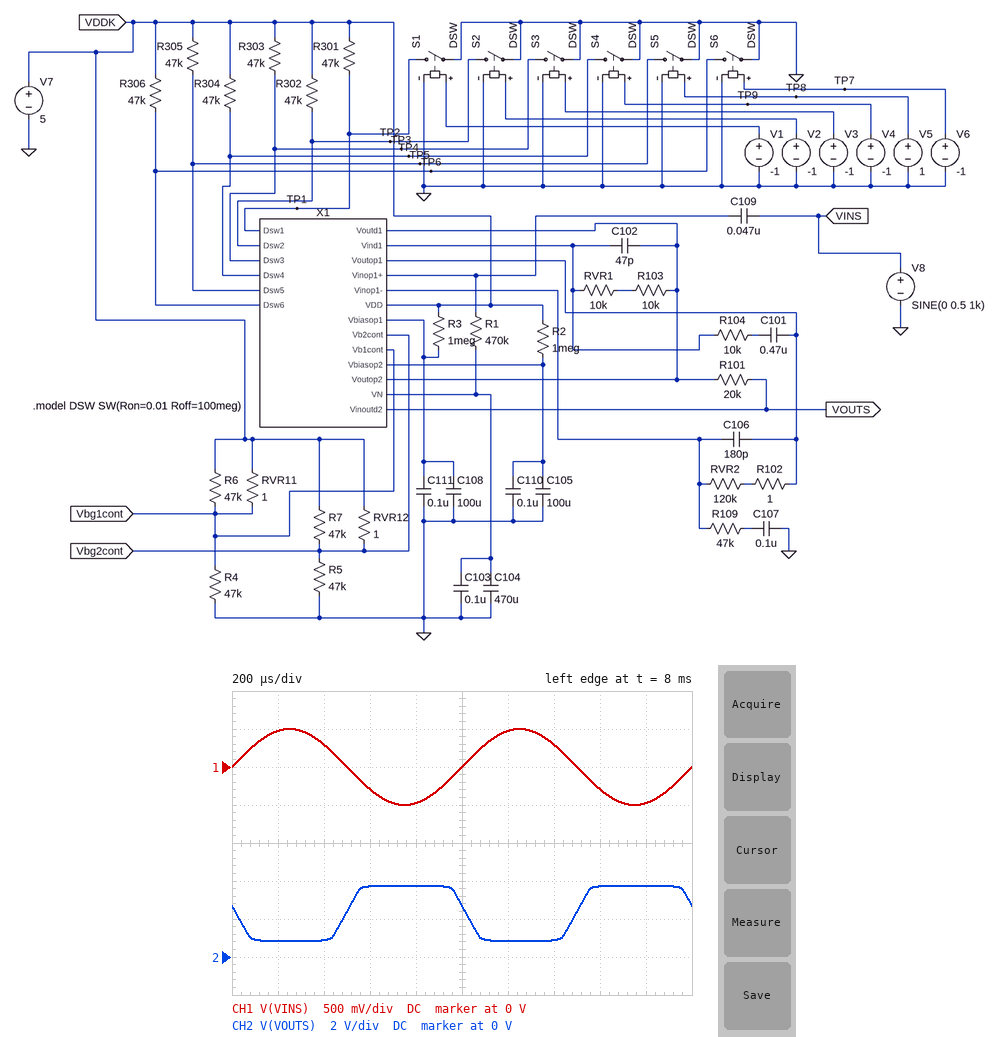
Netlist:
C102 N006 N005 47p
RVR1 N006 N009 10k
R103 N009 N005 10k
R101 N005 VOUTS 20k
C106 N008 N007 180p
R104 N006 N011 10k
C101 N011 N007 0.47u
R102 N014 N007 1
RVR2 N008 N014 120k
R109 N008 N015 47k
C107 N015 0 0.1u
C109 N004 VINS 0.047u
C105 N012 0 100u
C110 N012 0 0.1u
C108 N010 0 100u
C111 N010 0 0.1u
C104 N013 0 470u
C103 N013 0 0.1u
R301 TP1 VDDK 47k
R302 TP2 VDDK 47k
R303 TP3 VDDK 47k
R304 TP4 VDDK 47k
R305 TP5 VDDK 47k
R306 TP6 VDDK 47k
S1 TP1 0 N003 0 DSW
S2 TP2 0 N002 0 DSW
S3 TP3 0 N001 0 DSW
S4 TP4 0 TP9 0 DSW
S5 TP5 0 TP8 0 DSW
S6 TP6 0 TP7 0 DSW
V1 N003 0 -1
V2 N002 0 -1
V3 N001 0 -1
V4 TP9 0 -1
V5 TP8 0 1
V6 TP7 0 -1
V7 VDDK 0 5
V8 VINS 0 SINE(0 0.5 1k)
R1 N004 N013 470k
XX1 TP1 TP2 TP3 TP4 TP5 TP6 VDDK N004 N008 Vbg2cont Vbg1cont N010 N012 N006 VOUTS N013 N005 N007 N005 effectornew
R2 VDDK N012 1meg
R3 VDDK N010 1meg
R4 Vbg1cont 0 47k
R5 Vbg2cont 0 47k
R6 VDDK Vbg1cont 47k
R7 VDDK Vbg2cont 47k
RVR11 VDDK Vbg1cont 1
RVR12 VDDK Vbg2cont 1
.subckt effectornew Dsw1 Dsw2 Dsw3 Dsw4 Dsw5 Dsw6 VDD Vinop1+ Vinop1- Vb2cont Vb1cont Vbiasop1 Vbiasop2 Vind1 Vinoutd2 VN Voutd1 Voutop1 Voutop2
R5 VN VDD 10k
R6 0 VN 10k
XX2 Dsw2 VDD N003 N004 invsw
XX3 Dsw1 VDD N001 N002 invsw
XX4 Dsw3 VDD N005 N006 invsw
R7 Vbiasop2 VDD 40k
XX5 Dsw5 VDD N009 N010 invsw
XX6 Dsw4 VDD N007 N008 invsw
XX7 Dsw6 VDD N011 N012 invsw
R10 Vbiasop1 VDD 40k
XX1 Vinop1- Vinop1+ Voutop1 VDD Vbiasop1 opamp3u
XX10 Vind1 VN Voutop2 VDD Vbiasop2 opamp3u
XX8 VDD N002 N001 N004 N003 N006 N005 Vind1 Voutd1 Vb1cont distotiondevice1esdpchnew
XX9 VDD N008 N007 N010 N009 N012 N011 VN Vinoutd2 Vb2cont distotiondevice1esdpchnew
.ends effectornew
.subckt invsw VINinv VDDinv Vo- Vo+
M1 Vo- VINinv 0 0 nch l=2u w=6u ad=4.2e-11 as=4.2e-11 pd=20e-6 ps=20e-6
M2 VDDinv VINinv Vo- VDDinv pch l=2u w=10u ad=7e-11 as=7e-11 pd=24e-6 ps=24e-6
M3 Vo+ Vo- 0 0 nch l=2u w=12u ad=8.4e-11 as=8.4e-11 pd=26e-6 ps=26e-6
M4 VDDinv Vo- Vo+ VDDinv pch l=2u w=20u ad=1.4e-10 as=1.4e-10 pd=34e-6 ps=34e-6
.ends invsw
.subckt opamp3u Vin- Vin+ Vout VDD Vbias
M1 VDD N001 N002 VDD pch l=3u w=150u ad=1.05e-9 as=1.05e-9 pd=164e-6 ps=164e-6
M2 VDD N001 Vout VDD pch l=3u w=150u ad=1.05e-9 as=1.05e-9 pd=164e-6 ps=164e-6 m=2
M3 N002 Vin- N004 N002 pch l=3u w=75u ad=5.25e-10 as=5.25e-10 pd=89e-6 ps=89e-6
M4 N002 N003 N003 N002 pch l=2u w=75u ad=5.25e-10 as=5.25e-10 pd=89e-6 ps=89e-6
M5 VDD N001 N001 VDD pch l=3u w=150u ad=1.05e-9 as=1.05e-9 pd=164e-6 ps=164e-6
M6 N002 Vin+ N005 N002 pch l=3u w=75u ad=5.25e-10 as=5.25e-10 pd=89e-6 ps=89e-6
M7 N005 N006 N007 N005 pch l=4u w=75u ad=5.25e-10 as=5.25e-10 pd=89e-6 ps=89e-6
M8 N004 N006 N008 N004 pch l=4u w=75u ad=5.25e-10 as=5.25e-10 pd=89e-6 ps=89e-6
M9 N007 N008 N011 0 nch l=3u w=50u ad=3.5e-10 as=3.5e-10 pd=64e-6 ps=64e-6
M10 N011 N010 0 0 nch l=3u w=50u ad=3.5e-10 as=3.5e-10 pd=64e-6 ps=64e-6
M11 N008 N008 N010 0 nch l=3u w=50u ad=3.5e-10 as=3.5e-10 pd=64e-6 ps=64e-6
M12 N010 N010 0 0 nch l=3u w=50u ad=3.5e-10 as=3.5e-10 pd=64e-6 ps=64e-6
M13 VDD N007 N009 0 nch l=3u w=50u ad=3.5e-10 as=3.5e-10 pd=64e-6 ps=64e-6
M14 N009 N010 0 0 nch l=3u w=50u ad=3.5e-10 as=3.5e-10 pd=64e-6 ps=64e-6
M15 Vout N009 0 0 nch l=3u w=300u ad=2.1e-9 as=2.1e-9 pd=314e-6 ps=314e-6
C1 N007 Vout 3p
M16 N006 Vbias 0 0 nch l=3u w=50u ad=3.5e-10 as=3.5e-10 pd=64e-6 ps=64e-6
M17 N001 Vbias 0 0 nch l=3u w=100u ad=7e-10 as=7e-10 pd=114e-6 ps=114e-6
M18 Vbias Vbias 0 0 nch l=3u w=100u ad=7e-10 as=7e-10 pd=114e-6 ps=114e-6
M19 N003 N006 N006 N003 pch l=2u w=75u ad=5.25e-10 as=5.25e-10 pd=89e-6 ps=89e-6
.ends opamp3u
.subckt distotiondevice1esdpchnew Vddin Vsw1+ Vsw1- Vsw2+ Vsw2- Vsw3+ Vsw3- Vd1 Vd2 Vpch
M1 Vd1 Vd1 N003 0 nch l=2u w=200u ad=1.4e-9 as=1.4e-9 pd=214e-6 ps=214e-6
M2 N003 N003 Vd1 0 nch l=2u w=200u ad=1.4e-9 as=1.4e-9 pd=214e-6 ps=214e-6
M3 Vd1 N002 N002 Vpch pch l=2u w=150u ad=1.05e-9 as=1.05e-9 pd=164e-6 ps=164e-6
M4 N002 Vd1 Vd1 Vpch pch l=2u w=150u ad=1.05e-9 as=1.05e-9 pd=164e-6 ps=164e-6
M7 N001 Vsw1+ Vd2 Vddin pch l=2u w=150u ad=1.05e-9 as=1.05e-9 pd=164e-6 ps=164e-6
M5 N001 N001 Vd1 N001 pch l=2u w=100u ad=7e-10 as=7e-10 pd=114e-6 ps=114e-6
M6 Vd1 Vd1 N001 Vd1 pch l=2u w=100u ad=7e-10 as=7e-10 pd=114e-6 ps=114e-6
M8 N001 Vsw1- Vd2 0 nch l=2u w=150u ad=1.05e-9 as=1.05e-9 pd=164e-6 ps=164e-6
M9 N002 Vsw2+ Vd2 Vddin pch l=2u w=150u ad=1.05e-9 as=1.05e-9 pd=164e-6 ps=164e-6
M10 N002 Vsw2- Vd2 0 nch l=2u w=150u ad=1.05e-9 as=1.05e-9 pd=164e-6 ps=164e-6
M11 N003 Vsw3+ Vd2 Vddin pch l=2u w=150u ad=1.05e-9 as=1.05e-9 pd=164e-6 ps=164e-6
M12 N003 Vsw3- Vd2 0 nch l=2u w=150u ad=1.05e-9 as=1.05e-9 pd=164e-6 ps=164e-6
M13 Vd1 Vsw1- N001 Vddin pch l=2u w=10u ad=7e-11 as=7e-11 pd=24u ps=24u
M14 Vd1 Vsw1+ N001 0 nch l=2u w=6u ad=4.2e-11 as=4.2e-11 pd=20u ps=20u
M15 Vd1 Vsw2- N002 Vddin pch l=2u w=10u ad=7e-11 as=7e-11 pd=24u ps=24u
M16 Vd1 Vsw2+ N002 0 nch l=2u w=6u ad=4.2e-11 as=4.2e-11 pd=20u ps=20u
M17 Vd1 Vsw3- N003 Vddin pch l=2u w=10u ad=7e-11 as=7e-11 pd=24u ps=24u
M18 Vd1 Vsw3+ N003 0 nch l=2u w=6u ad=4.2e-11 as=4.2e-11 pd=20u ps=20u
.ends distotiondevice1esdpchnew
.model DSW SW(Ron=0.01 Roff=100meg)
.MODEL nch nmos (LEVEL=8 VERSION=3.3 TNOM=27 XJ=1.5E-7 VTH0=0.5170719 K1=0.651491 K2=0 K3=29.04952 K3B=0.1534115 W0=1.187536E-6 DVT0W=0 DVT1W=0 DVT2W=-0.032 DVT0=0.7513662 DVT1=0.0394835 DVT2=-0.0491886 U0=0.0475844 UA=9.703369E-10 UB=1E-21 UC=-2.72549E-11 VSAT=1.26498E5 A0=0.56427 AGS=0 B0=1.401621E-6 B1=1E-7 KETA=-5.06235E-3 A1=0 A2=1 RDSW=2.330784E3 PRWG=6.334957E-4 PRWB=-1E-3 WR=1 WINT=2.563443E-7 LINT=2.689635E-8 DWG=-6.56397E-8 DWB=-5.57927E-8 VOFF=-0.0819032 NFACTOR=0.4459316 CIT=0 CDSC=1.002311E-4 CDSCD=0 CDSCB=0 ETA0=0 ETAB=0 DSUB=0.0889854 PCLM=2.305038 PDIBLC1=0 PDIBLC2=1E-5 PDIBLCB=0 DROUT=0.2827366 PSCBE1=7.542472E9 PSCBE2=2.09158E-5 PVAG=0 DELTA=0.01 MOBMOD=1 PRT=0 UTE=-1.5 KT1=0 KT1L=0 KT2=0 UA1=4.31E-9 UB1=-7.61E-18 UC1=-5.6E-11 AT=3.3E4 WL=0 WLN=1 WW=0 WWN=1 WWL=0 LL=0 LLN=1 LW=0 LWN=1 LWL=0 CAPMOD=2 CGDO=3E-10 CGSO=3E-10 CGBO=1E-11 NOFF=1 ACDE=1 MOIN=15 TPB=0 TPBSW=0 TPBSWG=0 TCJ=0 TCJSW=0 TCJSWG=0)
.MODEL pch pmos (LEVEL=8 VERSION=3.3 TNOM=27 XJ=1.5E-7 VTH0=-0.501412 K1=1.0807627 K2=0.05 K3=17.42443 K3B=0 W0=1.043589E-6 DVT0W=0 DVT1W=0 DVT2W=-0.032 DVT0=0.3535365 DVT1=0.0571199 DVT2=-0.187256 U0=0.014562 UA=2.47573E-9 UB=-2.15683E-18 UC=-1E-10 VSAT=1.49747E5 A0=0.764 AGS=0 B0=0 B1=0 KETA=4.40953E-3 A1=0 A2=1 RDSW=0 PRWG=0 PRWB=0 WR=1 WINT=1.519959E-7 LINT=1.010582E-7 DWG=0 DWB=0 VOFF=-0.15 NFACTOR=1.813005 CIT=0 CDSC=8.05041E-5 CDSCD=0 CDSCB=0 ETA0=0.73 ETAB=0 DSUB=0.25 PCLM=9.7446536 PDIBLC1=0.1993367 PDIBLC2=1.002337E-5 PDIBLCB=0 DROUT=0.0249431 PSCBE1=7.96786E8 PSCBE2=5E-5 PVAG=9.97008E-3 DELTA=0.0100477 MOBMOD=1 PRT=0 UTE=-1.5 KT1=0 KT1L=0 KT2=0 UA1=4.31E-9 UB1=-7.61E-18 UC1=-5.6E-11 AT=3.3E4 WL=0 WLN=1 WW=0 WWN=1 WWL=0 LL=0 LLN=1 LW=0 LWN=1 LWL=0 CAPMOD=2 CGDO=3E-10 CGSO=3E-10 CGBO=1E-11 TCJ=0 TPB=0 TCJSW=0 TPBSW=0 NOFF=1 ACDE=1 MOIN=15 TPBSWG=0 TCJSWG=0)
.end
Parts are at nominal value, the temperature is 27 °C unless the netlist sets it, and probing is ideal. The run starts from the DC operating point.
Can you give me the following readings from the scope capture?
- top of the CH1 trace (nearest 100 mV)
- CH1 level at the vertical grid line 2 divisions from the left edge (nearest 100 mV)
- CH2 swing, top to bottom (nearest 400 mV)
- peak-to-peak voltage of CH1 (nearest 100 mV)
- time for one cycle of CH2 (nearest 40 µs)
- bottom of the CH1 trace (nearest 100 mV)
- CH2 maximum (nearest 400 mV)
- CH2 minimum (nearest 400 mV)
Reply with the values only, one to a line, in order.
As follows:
500 mV
300 mV
2.8 V
1.0 V
1.00 ms
-500 mV
3.6 V
800 mV
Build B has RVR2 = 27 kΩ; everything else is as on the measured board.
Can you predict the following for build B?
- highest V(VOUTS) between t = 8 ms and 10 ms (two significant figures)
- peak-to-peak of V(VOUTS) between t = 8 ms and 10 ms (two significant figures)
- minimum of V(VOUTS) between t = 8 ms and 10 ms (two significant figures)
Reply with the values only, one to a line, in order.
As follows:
3.7 V
2.7 V
990 mV
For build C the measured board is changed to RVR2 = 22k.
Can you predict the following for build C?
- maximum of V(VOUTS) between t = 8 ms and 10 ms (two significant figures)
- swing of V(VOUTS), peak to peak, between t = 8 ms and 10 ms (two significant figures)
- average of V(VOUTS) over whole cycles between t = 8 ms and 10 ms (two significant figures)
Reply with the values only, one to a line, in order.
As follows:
3.7 V
2.6 V
2.5 V
